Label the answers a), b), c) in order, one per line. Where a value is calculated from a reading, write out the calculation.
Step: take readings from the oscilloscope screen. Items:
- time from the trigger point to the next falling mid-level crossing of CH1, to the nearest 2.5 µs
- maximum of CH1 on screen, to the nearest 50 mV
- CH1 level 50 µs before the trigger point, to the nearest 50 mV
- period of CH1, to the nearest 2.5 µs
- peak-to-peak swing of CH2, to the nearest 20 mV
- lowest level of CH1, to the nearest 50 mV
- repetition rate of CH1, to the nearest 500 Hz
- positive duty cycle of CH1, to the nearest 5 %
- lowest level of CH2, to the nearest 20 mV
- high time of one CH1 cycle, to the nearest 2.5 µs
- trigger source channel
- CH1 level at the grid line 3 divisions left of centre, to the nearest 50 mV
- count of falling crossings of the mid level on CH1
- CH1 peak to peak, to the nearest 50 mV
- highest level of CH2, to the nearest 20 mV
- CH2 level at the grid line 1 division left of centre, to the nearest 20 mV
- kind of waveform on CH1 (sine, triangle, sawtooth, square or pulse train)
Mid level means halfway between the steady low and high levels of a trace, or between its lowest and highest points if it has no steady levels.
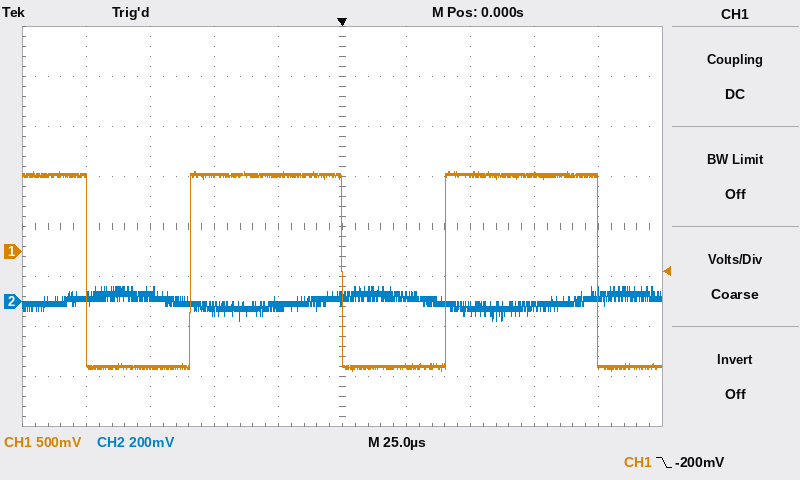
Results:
a) 100.0 µs
b) 800 mV
c) 750 mV
d) 100.0 µs
e) 60 mV − (-80 mV) = 140 mV
f) -1.20 V
g) 1 / 100.0 µs ≈ 10.0 kHz
h) 60.0 µs / 100.0 µs ≈ 60 %
i) -80 mV
j) 60.0 µs
k) CH1
l) -1.15 V
m) 3
n) 800 mV − (-1.20 V) = 2.00 V
o) 60 mV
p) -20 mV
q) pulse train
